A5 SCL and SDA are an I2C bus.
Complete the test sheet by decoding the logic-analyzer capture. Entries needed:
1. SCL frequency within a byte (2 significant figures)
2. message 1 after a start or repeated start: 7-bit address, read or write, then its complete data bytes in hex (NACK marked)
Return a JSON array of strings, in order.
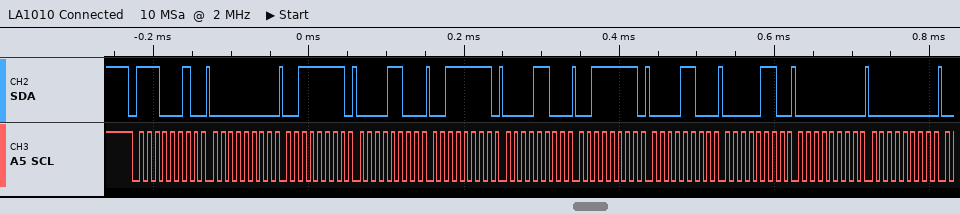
["100 kHz", "0x71 write: 00 3F 0C 3F 0C 3F 0C 06 00 00"]
